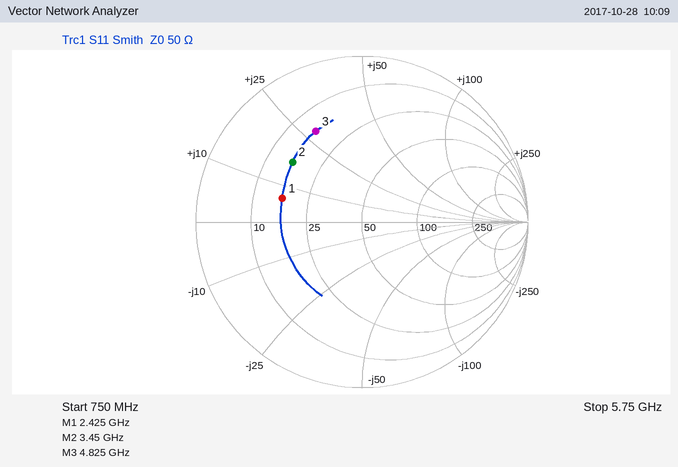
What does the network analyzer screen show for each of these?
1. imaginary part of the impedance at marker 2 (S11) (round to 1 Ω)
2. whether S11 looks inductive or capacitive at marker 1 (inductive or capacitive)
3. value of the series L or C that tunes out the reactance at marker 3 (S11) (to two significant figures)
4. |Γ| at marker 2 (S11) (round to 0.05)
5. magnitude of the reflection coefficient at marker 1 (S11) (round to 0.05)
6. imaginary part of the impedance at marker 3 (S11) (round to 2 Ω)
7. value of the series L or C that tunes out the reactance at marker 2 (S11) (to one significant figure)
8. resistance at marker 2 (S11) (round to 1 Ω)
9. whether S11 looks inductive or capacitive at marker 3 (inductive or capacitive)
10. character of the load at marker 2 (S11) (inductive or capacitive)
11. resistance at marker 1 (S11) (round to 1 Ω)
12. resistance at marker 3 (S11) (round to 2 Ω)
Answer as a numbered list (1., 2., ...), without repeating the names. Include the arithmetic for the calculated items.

1. +17 Ω
2. inductive
3. C = 1/(2π × 4.825 GHz × 28 Ω) ≈ 1.2 pF
4. 0.55
5. 0.50
6. +28 Ω
7. C = 1/(2π × 3.45 GHz × 17 Ω) ≈ 3 pF
8. 16 Ω
9. inductive
10. inductive
11. 17 Ω
12. 16 Ω
